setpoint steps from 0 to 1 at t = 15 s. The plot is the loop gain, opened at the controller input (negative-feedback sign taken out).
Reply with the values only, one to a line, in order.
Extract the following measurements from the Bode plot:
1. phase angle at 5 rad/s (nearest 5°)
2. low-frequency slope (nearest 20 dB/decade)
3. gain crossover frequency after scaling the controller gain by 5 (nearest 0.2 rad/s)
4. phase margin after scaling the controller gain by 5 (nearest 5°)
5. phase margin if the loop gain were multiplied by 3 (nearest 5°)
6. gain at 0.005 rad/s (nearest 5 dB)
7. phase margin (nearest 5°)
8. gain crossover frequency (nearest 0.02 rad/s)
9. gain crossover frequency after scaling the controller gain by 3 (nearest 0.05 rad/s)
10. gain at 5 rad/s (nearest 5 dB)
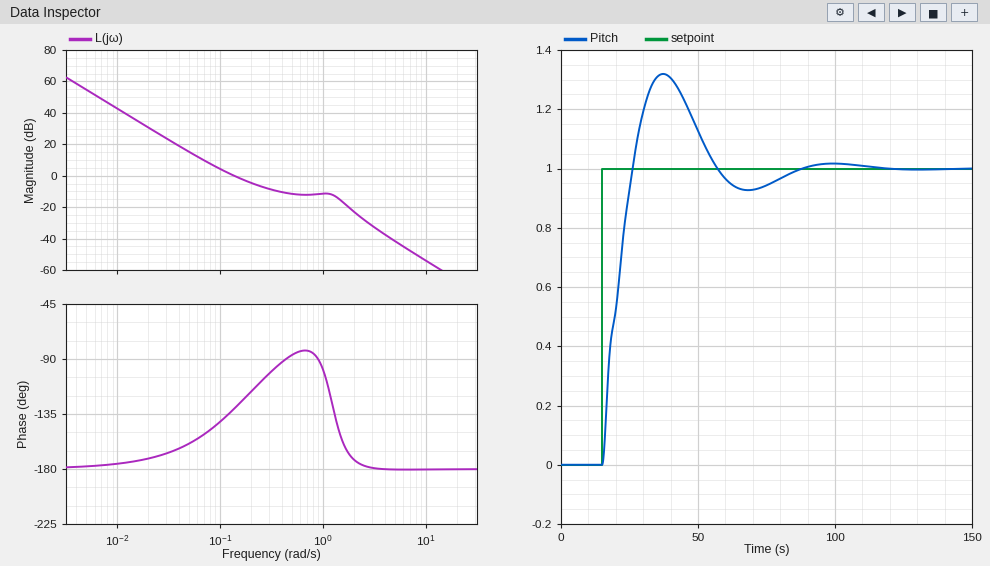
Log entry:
-180°
-40 dB/decade
1.4 rad/s
35°
85°
55 dB
50°
0.14 rad/s
0.35 rad/s
-40 dB
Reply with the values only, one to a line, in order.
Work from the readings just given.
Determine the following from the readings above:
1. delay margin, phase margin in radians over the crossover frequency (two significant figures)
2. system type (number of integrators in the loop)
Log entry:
6.2 s
2
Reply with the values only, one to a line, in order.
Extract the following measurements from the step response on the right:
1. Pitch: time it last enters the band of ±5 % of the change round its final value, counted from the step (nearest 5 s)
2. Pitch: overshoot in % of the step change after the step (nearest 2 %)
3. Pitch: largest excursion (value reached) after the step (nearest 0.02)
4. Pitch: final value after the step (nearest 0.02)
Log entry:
60 s
32 %
1.32
1.00
